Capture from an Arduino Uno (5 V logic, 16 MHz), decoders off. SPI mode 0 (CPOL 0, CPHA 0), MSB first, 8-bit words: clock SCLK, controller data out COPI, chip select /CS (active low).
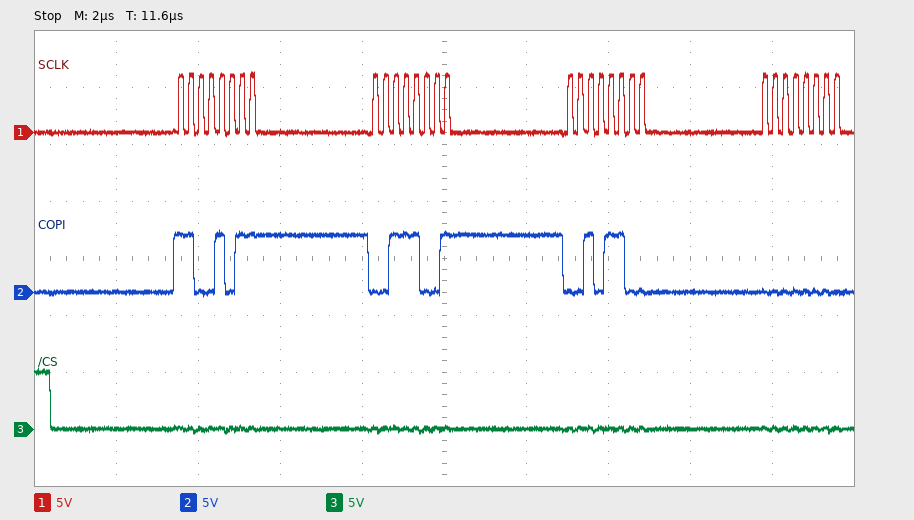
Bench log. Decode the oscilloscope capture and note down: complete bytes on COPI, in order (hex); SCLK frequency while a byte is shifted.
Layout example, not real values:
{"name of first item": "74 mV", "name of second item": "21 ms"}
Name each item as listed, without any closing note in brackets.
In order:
{"complete bytes on COPI, in order": "CB 39 2C 00", "SCLK frequency while a byte is shifted": "4 MHz"}
